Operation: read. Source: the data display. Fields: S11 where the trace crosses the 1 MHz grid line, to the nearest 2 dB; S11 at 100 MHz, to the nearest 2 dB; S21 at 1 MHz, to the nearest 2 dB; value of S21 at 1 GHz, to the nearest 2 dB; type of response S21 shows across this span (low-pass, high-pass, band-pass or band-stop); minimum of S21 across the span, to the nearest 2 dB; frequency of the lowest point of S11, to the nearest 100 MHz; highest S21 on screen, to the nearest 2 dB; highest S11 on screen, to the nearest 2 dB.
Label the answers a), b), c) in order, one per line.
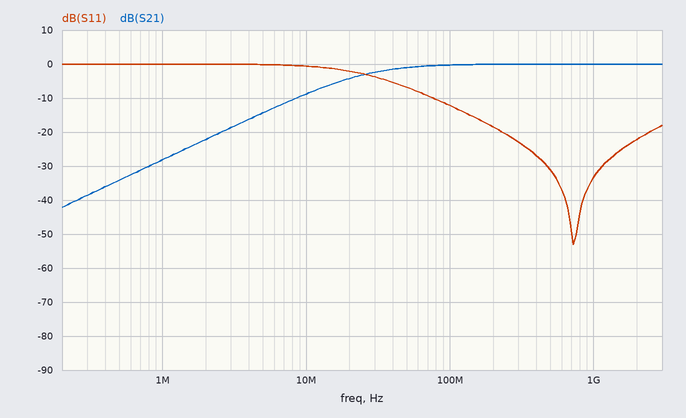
a) 0 dB
b) -12 dB
c) -28 dB
d) 0 dB
e) high-pass
f) -42 dB
g) 700 MHz
h) 0 dB
i) 0 dB
